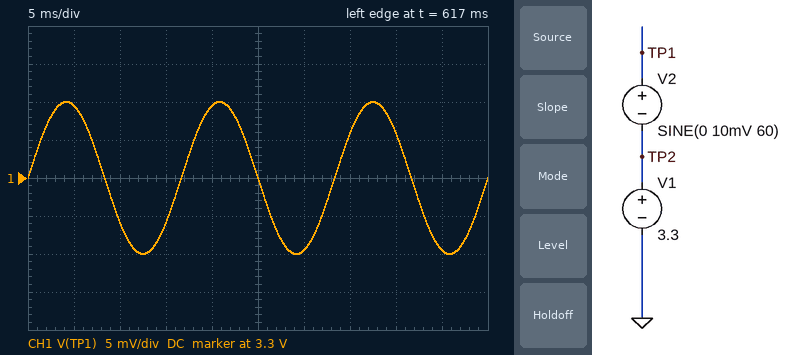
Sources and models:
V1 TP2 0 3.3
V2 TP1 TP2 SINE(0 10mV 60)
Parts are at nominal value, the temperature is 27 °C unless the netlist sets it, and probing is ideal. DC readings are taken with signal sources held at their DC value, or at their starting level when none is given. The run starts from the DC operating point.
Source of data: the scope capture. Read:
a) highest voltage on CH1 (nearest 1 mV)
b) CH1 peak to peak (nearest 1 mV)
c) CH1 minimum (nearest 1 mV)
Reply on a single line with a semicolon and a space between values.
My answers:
3.310 V; 20 mV; 3.290 V
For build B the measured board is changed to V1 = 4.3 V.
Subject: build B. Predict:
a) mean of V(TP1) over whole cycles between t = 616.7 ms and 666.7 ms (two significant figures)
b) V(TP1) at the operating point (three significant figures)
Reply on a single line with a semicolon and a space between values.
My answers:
4.3 V; 4.30 V
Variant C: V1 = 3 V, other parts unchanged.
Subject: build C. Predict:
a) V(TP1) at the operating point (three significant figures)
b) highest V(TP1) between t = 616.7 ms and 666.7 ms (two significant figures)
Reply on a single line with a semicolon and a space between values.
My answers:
3.00 V; 3.0 V
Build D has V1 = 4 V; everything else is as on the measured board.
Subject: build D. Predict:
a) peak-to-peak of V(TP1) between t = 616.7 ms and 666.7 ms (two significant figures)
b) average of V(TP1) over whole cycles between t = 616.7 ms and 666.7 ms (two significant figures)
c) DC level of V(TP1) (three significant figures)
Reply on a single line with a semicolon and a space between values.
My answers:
20 mV; 4.0 V; 4.00 V
